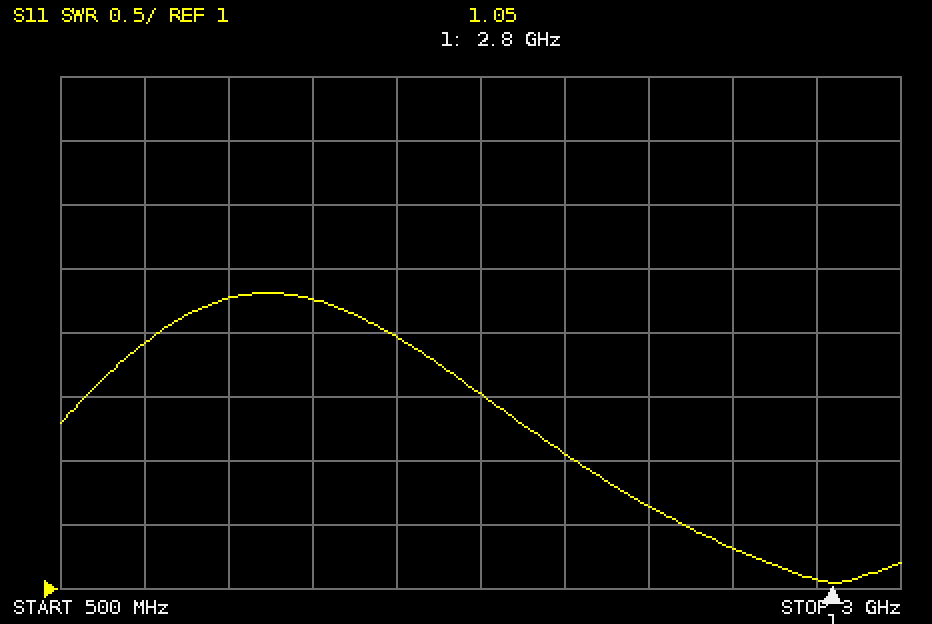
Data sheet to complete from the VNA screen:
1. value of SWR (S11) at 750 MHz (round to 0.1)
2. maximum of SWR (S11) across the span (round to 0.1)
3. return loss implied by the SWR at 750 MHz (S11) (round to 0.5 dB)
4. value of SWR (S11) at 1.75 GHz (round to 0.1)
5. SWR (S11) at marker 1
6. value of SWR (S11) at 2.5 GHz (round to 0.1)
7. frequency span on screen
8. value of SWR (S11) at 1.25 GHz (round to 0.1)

2.9
3.3
6.0 dB
2.5
1.05
1.3
2.5 GHz
3.3
